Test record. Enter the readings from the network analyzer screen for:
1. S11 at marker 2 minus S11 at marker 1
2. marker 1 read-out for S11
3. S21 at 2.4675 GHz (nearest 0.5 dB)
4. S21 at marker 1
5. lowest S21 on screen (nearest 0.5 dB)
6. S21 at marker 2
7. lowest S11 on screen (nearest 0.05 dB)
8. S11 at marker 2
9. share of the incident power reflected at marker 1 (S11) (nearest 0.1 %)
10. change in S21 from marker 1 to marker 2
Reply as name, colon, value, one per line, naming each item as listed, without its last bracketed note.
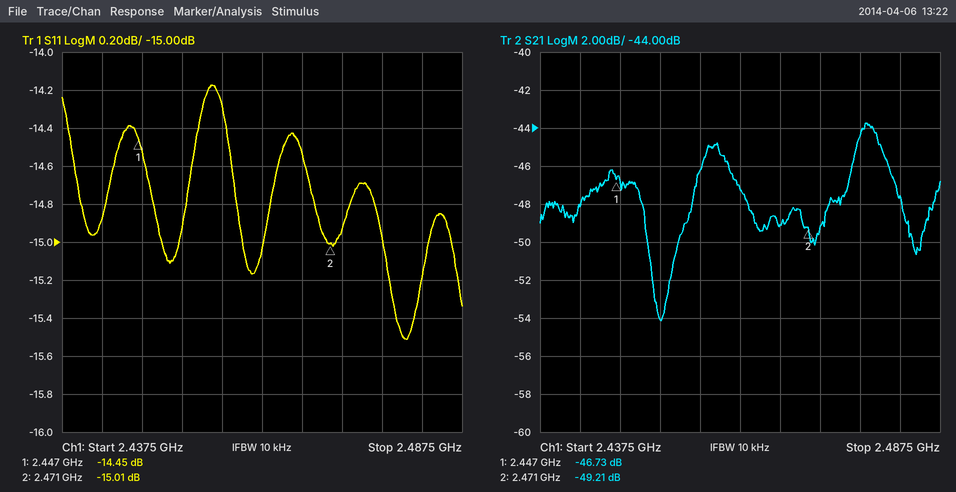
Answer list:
S11 at marker 2 minus S11 at marker 1: -0.56 dB
marker 1 read-out for S11: -14.45 dB
S21 at 2.4675 GHz: -49.0 dB
S21 at marker 1: -46.73 dB
lowest S21 on screen: -54.0 dB
S21 at marker 2: -49.21 dB
lowest S11 on screen: -15.50 dB
S11 at marker 2: -15.01 dB
share of the incident power reflected at marker 1 (S11): 3.6 %
change in S21 from marker 1 to marker 2: -2.48 dB
